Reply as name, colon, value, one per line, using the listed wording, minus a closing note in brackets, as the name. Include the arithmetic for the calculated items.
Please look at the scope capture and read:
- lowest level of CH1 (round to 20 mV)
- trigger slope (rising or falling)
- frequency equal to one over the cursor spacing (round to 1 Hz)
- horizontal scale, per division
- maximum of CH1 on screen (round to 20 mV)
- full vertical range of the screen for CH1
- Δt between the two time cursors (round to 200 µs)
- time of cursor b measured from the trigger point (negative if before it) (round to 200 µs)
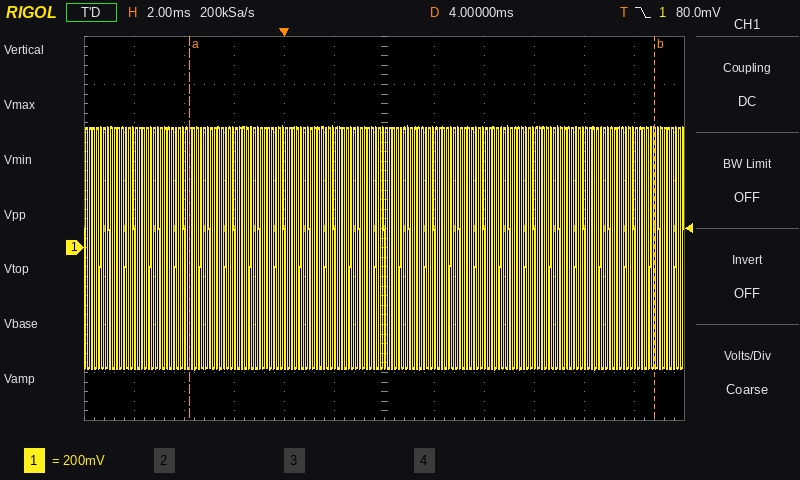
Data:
lowest level of CH1: -500 mV
trigger slope: falling
frequency equal to one over the cursor spacing: 1 / 18.6 ms ≈ 54 Hz
horizontal scale, per division: 2 ms
maximum of CH1 on screen: 500 mV
full vertical range of the screen for CH1: 1.6 V
Δt between the two time cursors: 18.6 ms
time of cursor b measured from the trigger point (negative if before it): +14.8 ms
